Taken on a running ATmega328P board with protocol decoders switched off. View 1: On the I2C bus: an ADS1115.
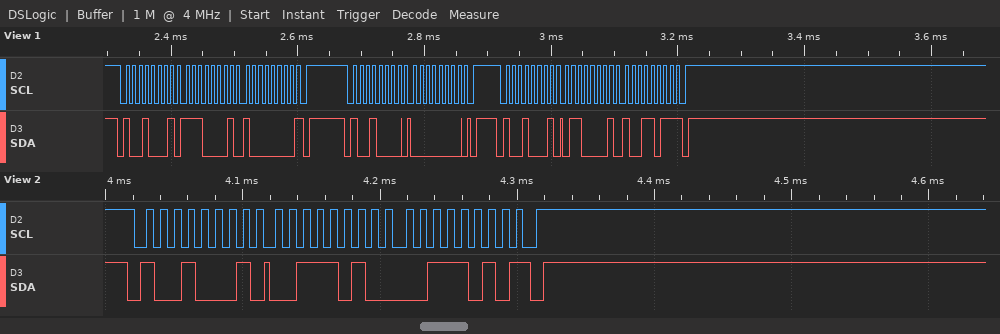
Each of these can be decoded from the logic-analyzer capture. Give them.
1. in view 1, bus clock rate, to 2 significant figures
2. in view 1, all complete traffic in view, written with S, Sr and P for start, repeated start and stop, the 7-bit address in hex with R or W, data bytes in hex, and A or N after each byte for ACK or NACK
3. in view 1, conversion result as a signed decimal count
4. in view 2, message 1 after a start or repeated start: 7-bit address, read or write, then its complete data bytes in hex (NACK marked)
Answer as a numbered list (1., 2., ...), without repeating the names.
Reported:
1. 100 kHz
2. S 48R A E1 A 80 N P S 48W A 00 A P S 48R A 61 A 9B N P
3. 24987
4. 0x48 read: 3A 3A NACK
